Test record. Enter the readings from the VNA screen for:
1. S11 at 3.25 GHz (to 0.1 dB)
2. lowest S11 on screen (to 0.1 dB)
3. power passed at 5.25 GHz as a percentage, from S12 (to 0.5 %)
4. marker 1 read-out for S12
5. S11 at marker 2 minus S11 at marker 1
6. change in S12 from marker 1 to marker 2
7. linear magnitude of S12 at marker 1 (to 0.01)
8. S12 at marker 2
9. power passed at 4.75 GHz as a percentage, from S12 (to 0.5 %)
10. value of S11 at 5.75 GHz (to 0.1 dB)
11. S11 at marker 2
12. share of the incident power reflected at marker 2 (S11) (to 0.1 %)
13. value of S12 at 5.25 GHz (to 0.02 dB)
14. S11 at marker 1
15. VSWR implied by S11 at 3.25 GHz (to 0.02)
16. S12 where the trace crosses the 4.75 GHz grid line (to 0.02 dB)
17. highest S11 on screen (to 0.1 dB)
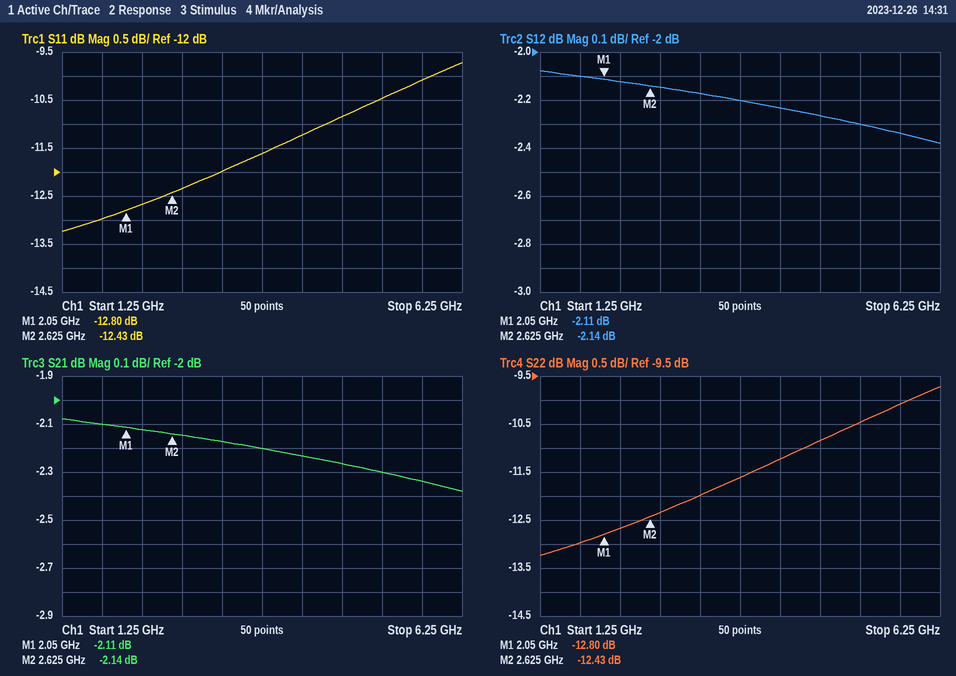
-12.0 dB
-13.2 dB
59.0 %
-2.11 dB
0.37 dB
-0.03 dB
0.78
-2.14 dB
59.5 %
-10.1 dB
-12.43 dB
5.7 %
-2.30 dB
-12.80 dB
1.68
-2.26 dB
-9.7 dB
